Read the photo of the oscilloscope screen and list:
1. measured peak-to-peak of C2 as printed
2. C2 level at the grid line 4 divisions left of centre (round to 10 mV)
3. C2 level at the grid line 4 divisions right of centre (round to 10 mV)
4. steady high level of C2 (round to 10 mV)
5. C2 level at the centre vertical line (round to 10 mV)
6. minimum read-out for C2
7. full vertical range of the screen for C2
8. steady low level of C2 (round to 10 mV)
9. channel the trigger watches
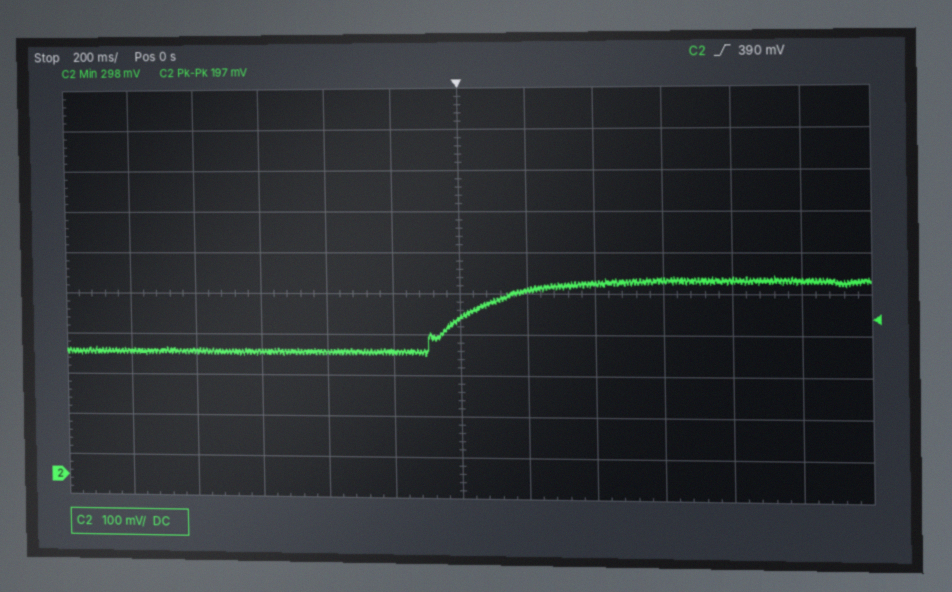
197 mV
310 mV
480 mV
480 mV
390 mV
298 mV
1 V
310 mV
C2
